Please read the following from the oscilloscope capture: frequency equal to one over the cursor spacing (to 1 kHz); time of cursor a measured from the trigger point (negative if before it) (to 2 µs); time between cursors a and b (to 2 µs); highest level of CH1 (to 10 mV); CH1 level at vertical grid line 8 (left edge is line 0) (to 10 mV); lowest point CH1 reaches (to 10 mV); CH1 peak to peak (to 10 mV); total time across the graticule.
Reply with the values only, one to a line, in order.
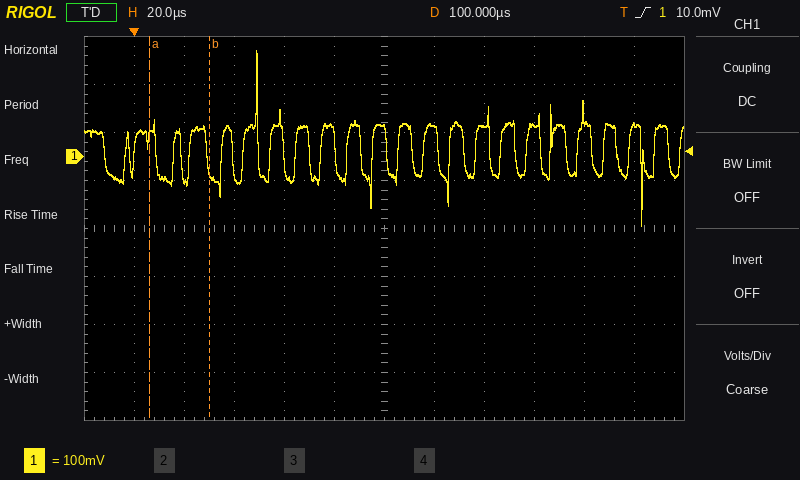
42 kHz
+6 µs
24 µs
220 mV
60 mV
-140 mV
360 mV
240 µs
